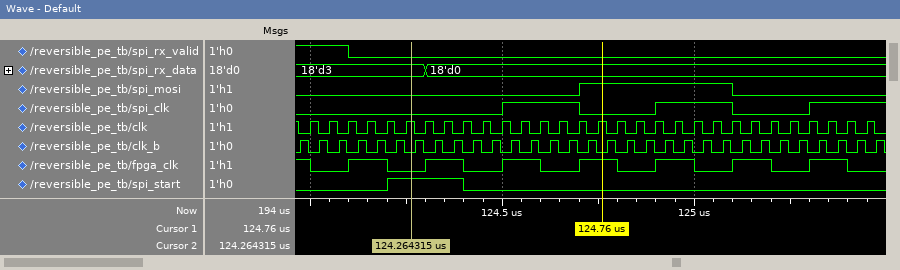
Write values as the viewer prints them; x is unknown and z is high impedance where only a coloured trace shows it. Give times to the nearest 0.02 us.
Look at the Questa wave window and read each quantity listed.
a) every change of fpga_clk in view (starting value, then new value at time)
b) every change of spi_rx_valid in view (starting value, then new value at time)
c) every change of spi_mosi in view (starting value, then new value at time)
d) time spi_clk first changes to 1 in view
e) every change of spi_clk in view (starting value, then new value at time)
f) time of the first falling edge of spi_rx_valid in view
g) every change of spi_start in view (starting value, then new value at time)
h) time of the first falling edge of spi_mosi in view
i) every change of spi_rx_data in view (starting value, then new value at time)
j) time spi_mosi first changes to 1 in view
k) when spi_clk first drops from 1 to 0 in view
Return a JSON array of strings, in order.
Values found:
["1, 0 at 124 us, 1 at 124.1 us, 0 at 124.2 us, 1 at 124.3 us, 0 at 124.4 us, 1 at 124.5 us, 0 at 124.6 us, 1 at 124.7 us, 0 at 124.8 us, 1 at 124.9 us, 0 at 125 us, 1 at 125.1 us, 0 at 125.2 us, 1 at 125.3 us, 0 at 125.4 us", "1, 0 at 124.1 us", "0, 1 at 124.7 us, 0 at 125.1 us", "124.5 us", "0, 1 at 124.5 us, 0 at 124.7 us, 1 at 124.9 us, 0 at 125.1 us, 1 at 125.3 us", "124.1 us", "0, 1 at 124.2 us, 0 at 124.4 us", "125.1 us", "18'd3, 18'd0 at 124.3 us", "124.7 us", "124.7 us"]
